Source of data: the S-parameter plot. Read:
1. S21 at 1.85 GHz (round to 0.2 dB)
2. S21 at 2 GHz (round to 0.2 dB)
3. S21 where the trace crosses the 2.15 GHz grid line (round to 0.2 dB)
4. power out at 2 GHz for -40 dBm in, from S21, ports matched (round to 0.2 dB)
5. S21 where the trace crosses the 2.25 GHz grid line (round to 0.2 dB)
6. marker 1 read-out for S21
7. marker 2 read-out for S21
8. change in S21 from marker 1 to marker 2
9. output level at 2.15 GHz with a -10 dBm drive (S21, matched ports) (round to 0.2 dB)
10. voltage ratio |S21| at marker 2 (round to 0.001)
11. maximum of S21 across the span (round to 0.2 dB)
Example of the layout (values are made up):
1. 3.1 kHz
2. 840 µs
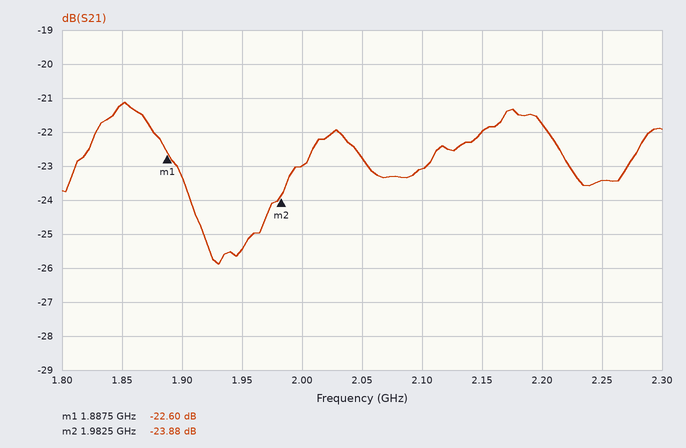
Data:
1. -21.2 dB
2. -23.0 dB
3. -22.0 dB
4. -63.0 dBm
5. -23.4 dB
6. -22.60 dB
7. -23.88 dB
8. -1.28 dB
9. -32.0 dBm
10. 0.064
11. -21.2 dB
